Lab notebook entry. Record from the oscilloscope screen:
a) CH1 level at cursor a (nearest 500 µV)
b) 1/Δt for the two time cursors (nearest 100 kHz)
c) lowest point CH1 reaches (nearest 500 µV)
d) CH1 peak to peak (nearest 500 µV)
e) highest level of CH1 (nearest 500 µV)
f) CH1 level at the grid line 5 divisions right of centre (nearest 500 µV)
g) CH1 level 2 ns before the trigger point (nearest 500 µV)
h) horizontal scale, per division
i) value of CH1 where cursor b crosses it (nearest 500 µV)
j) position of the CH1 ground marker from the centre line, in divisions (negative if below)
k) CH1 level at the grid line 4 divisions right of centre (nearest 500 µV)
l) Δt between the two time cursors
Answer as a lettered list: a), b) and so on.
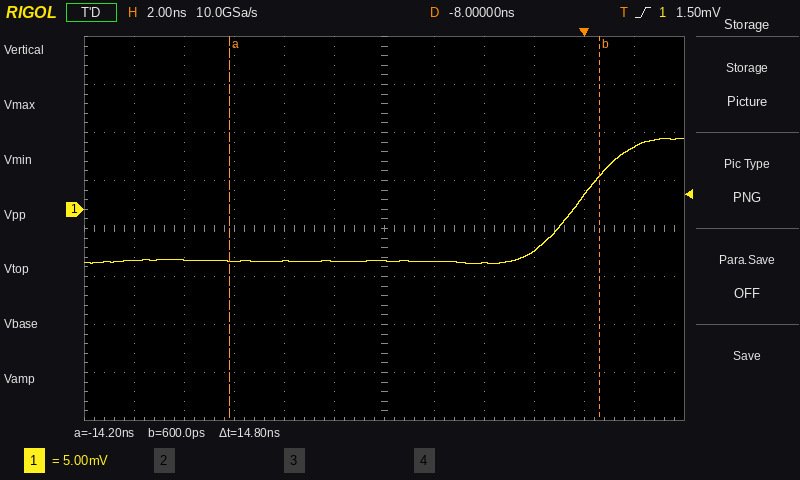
a) -5.5 mV
b) 67.6 MHz
c) -5.5 mV
d) 13.0 mV
e) 7.5 mV
f) 6.5 mV
g) -4.5 mV
h) 2 ns
i) 3.5 mV
j) +0.4 div
k) 1.5 mV
l) 14.8 ns
